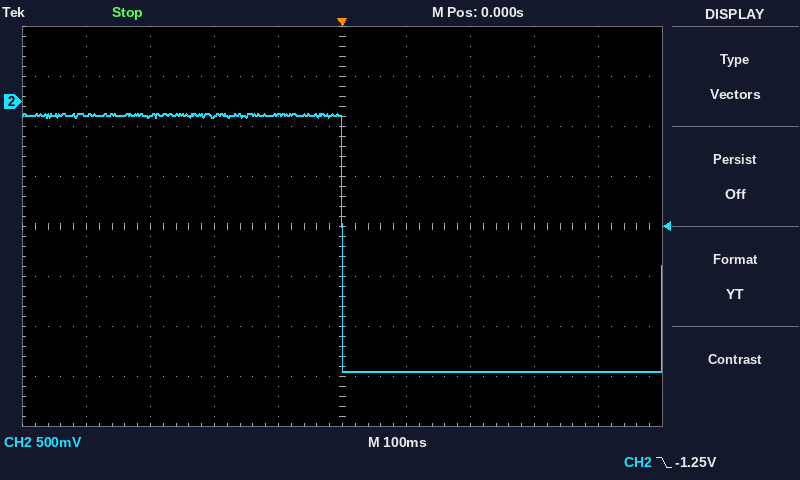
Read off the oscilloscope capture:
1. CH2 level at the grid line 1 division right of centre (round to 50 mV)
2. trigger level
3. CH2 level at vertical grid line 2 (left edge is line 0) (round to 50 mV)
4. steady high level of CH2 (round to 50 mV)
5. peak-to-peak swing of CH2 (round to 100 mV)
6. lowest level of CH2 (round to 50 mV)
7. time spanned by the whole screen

-2.70 V
-1.25 V
-150 mV
-150 mV
2.60 V
-2.70 V
1 s
